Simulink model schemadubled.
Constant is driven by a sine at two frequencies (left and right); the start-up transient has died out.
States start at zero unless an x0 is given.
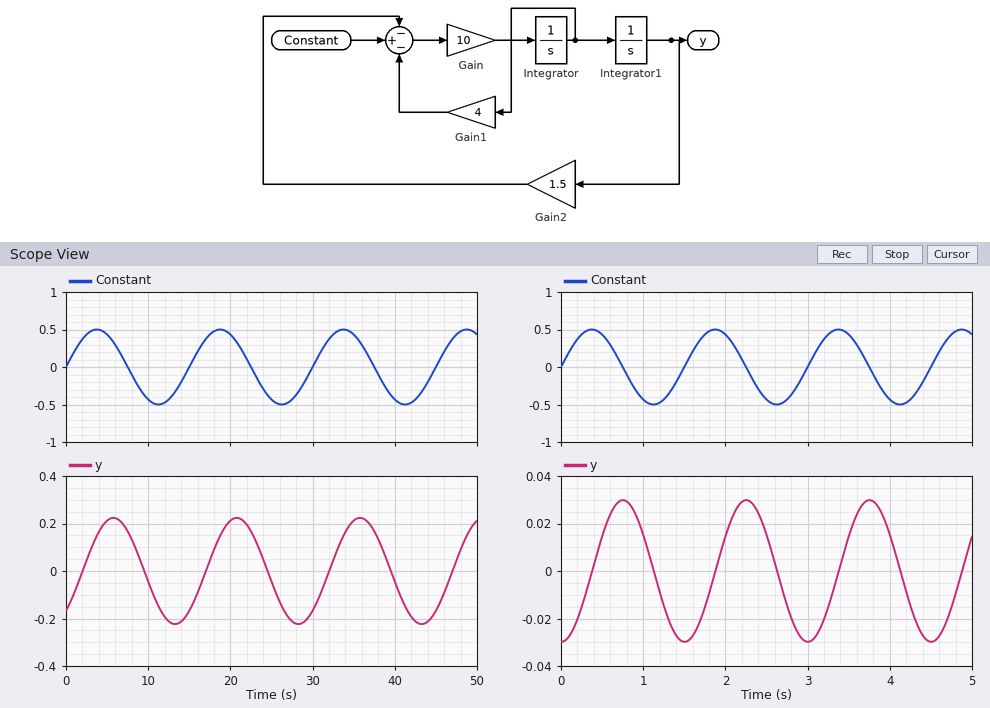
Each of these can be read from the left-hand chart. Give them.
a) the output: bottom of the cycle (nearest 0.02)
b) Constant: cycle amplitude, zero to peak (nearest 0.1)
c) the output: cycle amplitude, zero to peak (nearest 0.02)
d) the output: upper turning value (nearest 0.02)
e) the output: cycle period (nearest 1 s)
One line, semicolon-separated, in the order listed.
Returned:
-0.22; 0.5; 0.22; 0.22; 15 s
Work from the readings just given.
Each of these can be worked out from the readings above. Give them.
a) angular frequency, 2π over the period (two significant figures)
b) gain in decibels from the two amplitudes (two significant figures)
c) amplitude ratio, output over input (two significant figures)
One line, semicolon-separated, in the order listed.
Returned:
0.42 rad/s; -7.1 dB; 0.44
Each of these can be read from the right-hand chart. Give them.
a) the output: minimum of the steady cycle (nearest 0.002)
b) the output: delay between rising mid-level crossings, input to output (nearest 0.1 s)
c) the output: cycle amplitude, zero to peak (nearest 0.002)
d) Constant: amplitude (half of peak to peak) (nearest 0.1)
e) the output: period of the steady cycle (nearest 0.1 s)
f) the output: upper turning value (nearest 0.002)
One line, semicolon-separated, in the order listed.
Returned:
-0.030; 0.4 s; 0.030; 0.5; 1.5 s; 0.030
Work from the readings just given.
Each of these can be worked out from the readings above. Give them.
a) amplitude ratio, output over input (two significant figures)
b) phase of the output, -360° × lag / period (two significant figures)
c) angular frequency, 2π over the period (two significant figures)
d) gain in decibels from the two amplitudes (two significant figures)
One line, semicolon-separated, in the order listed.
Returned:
0.060; -96°; 4.2 rad/s; -24 dB
